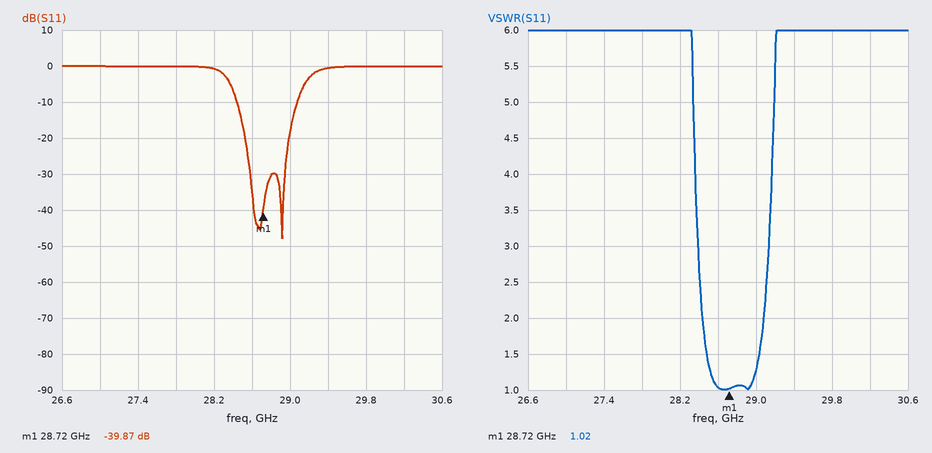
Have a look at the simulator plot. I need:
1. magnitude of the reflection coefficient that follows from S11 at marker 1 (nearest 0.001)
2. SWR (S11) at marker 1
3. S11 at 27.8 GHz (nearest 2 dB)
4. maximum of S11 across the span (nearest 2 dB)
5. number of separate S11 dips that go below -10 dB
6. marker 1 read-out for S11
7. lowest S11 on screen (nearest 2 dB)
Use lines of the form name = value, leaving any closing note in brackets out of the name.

magnitude of the reflection coefficient that follows from S11 at marker 1 = 0.010
SWR (S11) at marker 1 = 1.02
S11 at 27.8 GHz = 0 dB
maximum of S11 across the span = 0 dB
number of separate S11 dips that go below -10 dB = 2
marker 1 read-out for S11 = -39.87 dB
lowest S11 on screen = -48 dB
